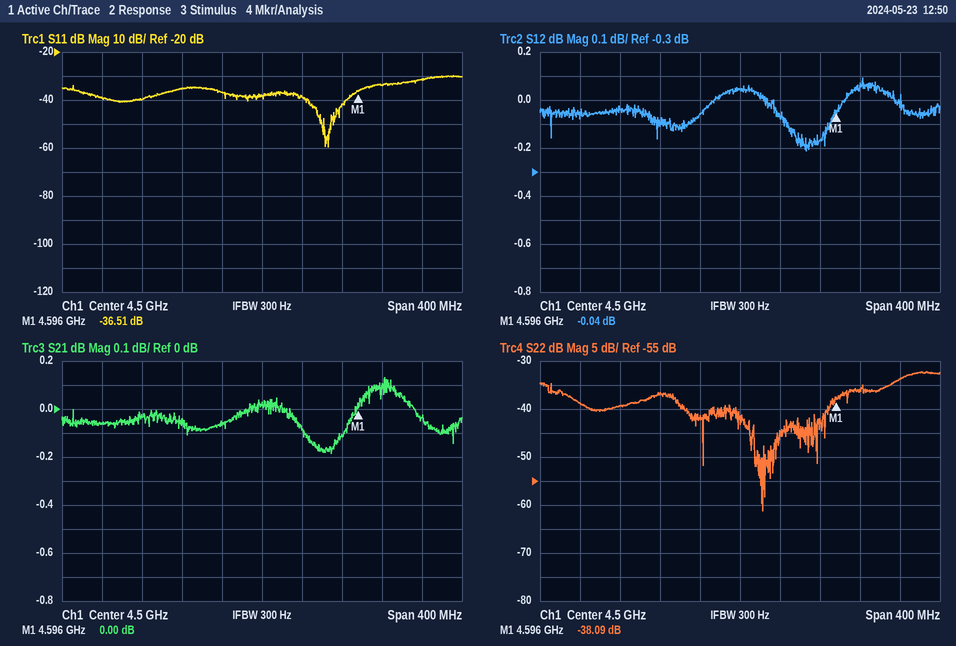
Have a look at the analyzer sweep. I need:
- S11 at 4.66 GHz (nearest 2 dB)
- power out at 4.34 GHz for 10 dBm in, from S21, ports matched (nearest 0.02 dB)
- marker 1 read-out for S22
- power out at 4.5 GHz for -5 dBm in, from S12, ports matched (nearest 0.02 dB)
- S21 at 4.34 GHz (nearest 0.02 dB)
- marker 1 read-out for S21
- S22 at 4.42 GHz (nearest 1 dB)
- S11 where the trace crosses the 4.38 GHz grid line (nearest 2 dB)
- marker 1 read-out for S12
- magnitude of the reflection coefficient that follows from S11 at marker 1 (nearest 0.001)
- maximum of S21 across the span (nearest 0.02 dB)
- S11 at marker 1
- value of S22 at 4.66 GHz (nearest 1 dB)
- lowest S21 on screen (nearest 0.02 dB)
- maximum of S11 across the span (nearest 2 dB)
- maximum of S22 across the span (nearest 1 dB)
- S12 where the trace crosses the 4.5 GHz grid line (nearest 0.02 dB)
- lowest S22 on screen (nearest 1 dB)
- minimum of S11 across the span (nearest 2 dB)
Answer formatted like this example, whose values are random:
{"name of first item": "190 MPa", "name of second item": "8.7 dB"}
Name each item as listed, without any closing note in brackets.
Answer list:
{"S11 at 4.66 GHz": "-32 dB", "power out at 4.34 GHz for 10 dBm in, from S21, ports matched": "9.94 dBm", "marker 1 read-out for S22": "-38.09 dB", "power out at 4.5 GHz for -5 dBm in, from S12, ports matched": "-4.96 dBm", "S21 at 4.34 GHz": "-0.06 dB", "marker 1 read-out for S21": "0.00 dB", "S22 at 4.42 GHz": "-37 dB", "S11 where the trace crosses the 4.38 GHz grid line": "-40 dB", "marker 1 read-out for S12": "-0.04 dB", "magnitude of the reflection coefficient that follows from S11 at marker 1": "0.015", "maximum of S21 across the span": "0.14 dB", "S11 at marker 1": "-36.51 dB", "value of S22 at 4.66 GHz": "-34 dB", "lowest S21 on screen": "-0.18 dB", "maximum of S11 across the span": "-30 dB", "maximum of S22 across the span": "-32 dB", "S12 where the trace crosses the 4.5 GHz grid line": "0.04 dB", "lowest S22 on screen": "-61 dB", "minimum of S11 across the span": "-60 dB"}
